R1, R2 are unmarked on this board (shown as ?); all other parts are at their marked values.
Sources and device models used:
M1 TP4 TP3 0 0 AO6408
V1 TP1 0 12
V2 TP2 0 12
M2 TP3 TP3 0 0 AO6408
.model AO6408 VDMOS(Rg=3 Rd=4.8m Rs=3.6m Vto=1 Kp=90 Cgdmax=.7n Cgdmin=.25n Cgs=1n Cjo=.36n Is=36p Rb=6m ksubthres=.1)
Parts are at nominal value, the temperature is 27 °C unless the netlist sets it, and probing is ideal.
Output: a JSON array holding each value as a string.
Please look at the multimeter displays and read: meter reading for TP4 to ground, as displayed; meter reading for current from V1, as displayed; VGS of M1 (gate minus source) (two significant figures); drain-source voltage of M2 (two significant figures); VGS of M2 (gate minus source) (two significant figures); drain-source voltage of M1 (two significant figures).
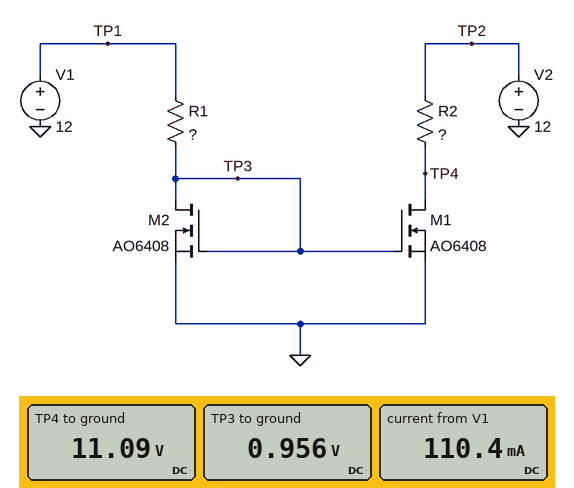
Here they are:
["11.09 V", "110.4 mA", "960 mV", "960 mV", "960 mV", "11 V"]
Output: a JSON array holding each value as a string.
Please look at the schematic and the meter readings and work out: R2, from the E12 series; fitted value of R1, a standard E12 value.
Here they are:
["8.2 Ω", "100 Ω"]
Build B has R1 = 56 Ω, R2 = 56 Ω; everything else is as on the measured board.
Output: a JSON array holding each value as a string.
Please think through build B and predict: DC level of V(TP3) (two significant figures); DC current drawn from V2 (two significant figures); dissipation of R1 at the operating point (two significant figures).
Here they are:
["990 mV", "200 mA", "2.2 W"]
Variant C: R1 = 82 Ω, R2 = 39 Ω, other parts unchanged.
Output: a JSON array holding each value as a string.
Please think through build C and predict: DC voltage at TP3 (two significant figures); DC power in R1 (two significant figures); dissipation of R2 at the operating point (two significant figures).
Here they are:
["970 mV", "1.5 W", "710 mW"]
